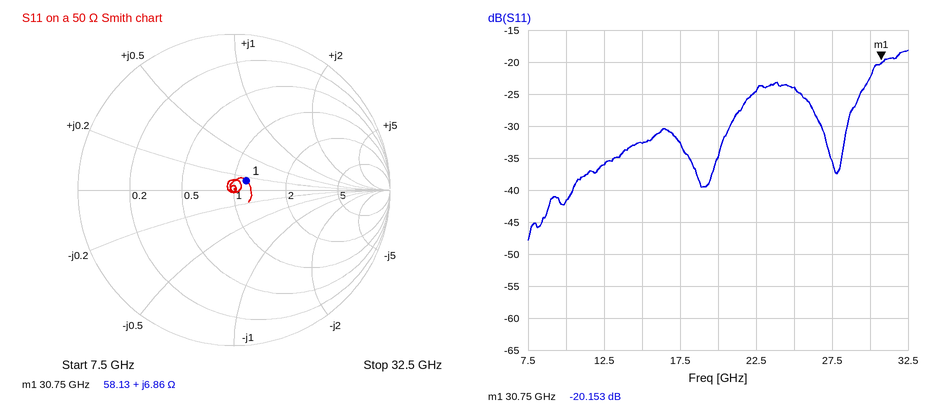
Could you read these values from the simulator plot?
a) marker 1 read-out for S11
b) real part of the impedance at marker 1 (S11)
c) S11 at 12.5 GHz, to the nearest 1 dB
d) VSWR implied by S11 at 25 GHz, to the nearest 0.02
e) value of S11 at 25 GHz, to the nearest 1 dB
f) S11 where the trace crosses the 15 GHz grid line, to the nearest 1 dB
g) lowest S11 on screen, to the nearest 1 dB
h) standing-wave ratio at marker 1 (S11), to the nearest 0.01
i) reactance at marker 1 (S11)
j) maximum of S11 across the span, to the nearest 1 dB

-20.153 dB
58.13 Ω
-36 dB
1.14
-24 dB
-33 dB
-48 dB
1.22
+6.86 Ω
-18 dB
